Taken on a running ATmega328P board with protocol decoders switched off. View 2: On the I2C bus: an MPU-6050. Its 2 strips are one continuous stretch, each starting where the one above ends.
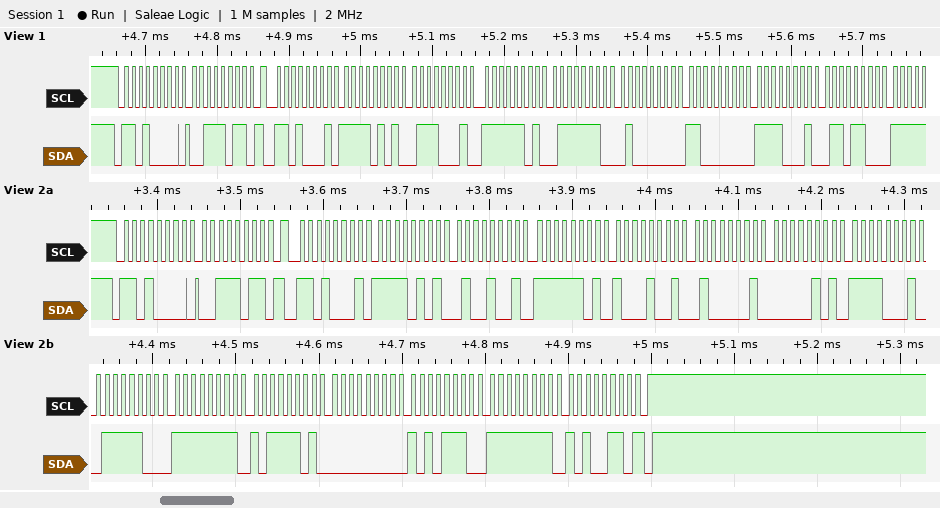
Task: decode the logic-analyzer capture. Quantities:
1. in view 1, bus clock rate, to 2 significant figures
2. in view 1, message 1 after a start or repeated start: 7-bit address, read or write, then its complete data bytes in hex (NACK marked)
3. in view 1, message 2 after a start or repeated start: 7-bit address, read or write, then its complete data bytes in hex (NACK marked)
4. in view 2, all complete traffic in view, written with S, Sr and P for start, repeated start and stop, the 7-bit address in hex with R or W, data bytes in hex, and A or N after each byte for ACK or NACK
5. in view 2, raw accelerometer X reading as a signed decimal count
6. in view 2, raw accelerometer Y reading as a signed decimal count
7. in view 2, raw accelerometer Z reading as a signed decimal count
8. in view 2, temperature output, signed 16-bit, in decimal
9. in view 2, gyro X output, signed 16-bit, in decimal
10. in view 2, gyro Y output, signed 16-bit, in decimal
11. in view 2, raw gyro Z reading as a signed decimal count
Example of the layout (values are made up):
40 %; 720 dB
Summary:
100 kHz; 0x68 write: 3B; 0x68 read: F5 71 FD 7E 40 C0 F1 6C; S 68W A 3B A Sr 68R A F5 A 49 A FD A 89 A 41 A 05 A F1 A 7C A FF A BD A 00 A AE A FF A A6 N P; -2743; -631; 16645; -3716; -67; 174; -90
